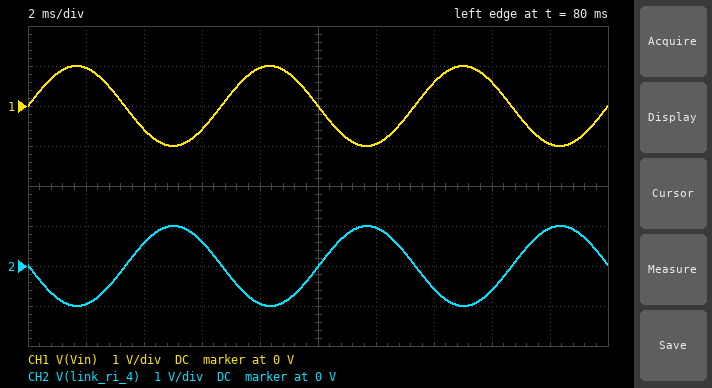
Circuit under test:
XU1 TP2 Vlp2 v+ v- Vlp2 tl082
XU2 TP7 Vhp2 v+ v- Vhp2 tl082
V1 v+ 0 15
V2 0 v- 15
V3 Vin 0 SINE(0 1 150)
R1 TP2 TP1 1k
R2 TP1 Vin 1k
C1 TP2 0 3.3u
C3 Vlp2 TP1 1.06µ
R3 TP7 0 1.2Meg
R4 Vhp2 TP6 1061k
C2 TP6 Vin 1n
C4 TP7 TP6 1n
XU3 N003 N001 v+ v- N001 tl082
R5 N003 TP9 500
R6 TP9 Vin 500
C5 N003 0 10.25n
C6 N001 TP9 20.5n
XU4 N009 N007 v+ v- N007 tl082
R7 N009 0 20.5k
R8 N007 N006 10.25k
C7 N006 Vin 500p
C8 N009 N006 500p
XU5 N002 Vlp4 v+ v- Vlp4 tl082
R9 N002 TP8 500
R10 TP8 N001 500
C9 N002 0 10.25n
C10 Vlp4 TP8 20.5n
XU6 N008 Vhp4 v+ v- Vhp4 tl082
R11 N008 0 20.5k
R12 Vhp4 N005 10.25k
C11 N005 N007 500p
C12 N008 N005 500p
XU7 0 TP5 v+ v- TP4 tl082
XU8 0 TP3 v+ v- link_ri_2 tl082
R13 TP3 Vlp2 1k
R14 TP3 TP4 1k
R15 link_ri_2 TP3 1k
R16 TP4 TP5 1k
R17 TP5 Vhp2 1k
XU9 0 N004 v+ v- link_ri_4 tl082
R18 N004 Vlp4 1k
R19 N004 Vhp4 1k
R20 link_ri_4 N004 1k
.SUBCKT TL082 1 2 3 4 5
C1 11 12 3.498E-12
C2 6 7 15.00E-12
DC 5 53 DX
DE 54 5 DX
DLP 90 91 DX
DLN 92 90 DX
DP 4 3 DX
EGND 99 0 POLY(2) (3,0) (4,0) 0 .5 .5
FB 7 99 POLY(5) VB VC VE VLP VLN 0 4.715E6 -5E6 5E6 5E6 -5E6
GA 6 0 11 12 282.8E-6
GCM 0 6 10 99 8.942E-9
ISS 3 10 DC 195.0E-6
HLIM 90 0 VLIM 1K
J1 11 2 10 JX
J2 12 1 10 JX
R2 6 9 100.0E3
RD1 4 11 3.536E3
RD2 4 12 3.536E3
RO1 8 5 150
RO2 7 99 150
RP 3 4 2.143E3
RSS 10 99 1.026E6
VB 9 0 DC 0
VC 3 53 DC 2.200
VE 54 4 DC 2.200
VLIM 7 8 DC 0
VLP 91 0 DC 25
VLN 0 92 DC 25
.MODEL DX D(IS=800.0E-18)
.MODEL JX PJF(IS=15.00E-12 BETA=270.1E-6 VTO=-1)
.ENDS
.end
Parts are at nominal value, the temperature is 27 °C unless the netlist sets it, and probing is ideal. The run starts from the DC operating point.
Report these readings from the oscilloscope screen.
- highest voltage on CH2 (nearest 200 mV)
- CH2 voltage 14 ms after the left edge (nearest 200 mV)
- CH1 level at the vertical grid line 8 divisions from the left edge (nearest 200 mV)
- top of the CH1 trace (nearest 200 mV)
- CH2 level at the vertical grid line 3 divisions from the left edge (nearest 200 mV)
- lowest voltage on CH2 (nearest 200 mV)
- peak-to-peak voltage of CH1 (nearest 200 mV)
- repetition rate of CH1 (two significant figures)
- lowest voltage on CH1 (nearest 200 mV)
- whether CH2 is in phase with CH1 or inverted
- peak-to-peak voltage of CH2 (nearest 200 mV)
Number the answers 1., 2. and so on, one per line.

1. 1.0 V
2. -600 mV
3. 600 mV
4. 1.0 V
5. 600 mV
6. -1.0 V
7. 2.0 V
8. 150 Hz
9. -1.0 V
10. inverted
11. 2.0 V
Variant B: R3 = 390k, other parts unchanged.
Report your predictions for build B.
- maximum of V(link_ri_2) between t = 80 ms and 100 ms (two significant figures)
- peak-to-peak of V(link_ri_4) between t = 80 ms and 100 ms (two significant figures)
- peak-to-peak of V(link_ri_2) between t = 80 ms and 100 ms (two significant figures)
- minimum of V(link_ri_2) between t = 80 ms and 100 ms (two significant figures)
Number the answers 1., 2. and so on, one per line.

1. 310 mV
2. 2.0 V
3. 620 mV
4. -310 mV
